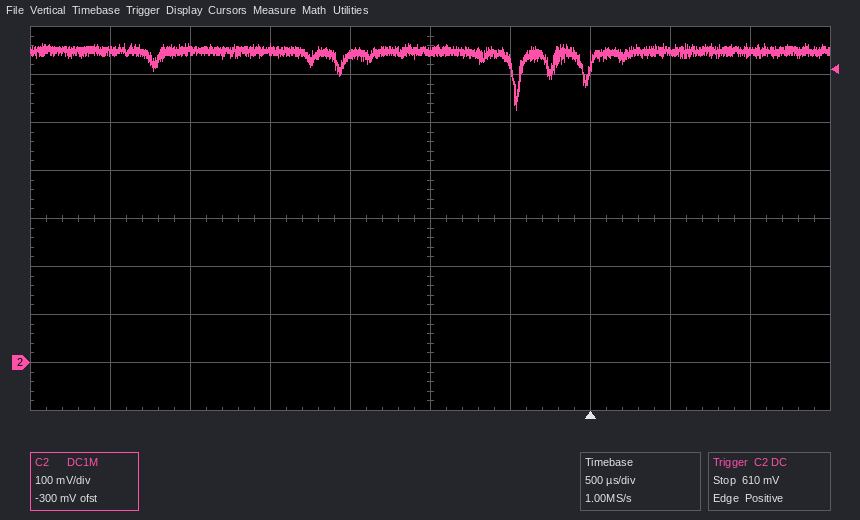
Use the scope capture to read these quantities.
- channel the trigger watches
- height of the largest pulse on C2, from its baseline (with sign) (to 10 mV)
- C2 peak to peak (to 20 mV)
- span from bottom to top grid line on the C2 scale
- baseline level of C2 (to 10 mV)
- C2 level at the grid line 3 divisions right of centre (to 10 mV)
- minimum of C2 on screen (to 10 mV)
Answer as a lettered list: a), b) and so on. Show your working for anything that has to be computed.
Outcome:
a) C2
b) 530 mV − (650 mV) = -120 mV
c) 140 mV
d) 800 mV
e) 650 mV
f) 650 mV
g) 530 mV
